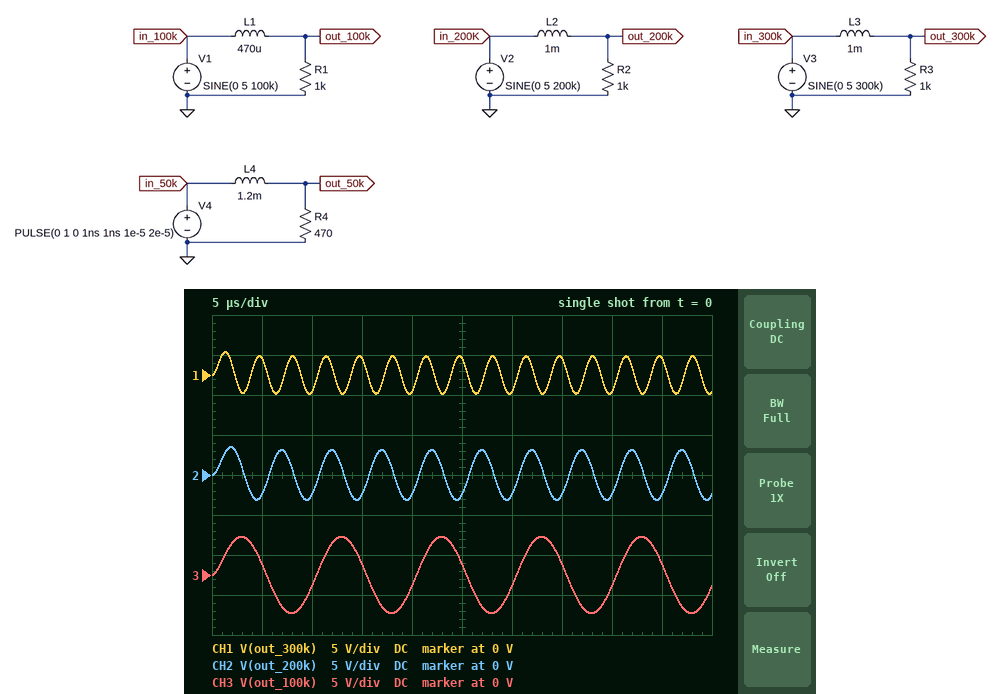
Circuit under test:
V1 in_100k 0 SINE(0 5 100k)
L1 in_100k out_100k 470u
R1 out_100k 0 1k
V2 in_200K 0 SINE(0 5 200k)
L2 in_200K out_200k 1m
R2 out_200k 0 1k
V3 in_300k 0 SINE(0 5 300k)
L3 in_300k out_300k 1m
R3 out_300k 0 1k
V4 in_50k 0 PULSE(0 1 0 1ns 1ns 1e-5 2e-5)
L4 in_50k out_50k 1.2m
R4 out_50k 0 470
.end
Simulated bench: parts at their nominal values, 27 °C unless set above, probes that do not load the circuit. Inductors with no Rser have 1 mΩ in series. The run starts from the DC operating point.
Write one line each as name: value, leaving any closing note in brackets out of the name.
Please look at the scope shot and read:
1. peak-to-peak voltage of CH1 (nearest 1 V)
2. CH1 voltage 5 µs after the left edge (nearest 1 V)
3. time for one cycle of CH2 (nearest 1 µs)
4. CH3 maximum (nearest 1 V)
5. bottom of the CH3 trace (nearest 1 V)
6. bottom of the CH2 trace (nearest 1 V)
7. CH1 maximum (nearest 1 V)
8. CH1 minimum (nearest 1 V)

peak-to-peak voltage of CH1: 5 V
CH1 voltage 5 µs after the left edge: 2 V
time for one cycle of CH2: 5 µs
CH3 maximum: 5 V
bottom of the CH3 trace: -5 V
bottom of the CH2 trace: -3 V
CH1 maximum: 3 V
CH1 minimum: -2 V
